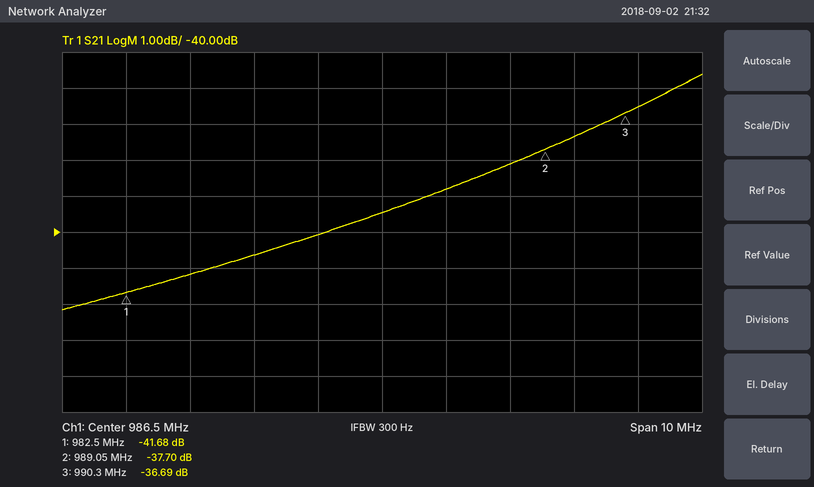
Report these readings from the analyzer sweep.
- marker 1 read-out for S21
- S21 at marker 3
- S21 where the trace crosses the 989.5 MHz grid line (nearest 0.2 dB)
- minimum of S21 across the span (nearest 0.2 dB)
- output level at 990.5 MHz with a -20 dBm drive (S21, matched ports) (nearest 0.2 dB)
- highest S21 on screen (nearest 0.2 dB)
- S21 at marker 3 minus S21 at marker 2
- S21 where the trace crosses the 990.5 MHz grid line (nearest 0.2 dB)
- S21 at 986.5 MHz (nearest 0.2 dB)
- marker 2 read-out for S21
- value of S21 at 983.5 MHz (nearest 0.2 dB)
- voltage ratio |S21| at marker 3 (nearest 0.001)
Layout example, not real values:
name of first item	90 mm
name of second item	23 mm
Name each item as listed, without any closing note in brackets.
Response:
marker 1 read-out for S21	-41.68 dB
S21 at marker 3	-36.69 dB
S21 where the trace crosses the 989.5 MHz grid line	-37.4 dB
minimum of S21 across the span	-42.2 dB
output level at 990.5 MHz with a -20 dBm drive (S21, matched ports)	-56.6 dBm
highest S21 on screen	-35.6 dB
S21 at marker 3 minus S21 at marker 2	1.01 dB
S21 where the trace crosses the 990.5 MHz grid line	-36.6 dB
S21 at 986.5 MHz	-39.4 dB
marker 2 read-out for S21	-37.70 dB
value of S21 at 983.5 MHz	-41.2 dB
voltage ratio |S21| at marker 3	0.015
